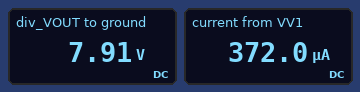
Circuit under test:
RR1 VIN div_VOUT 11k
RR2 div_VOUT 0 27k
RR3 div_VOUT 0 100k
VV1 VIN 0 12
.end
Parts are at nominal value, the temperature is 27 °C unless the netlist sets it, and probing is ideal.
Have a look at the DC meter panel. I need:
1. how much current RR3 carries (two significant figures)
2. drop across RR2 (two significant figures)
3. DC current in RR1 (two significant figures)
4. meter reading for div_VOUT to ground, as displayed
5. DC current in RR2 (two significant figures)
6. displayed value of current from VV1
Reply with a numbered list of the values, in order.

1. 79 µA
2. 7.9 V
3. 370 µA
4. 7.91 V
5. 290 µA
6. 372.0 µA
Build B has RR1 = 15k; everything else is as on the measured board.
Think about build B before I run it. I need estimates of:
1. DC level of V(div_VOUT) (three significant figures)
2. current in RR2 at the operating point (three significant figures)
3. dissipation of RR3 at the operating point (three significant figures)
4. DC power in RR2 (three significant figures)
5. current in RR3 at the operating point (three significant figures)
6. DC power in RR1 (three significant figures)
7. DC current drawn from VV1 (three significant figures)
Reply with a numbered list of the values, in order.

1. 7.04 V
2. 261 µA
3. 495 µW
4. 1.83 mW
5. 70.4 µA
6. 1.64 mW
7. 331 µA
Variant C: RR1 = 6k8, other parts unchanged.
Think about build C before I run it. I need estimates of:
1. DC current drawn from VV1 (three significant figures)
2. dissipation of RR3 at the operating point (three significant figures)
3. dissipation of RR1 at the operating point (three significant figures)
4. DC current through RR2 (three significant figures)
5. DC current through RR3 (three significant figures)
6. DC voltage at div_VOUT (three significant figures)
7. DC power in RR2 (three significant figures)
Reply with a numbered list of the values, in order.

1. 428 µA
2. 827 µW
3. 1.24 mW
4. 337 µA
5. 90.9 µA
6. 9.09 V
7. 3.06 mW
